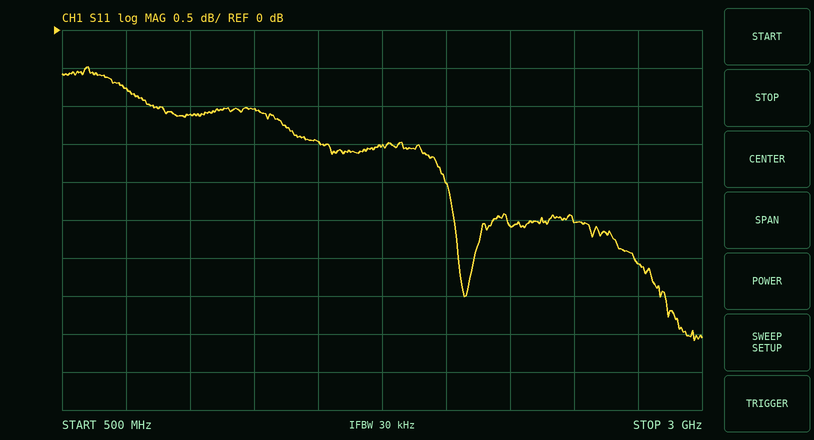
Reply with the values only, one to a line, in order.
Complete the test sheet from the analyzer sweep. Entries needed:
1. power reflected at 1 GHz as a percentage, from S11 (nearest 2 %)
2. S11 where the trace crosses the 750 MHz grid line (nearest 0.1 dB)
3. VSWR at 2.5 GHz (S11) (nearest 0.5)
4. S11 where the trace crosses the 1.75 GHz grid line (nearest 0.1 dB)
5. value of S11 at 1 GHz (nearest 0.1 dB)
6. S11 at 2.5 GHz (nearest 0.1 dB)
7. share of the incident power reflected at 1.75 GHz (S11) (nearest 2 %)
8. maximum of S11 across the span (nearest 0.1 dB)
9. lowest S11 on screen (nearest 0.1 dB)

78 %
-0.8 dB
7.0
-1.5 dB
-1.1 dB
-2.5 dB
70 %
-0.5 dB
-4.1 dB
